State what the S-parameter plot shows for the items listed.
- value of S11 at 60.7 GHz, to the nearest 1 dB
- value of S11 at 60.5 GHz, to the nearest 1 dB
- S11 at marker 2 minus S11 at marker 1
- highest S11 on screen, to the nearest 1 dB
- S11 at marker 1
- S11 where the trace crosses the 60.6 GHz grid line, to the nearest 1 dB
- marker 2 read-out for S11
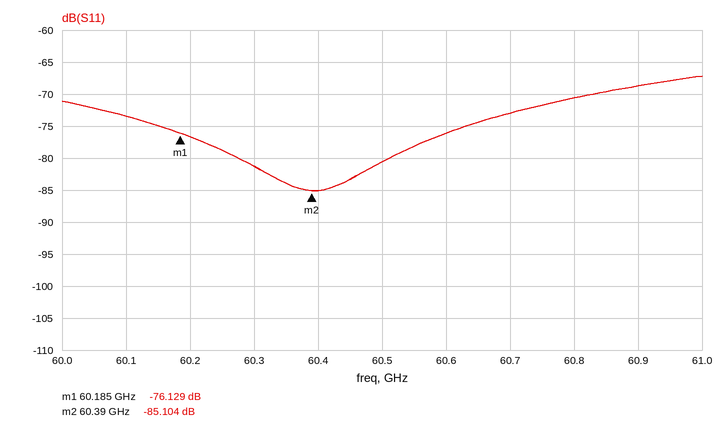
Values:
-73 dB
-81 dB
-8.975 dB
-67 dB
-76.129 dB
-76 dB
-85.104 dB
